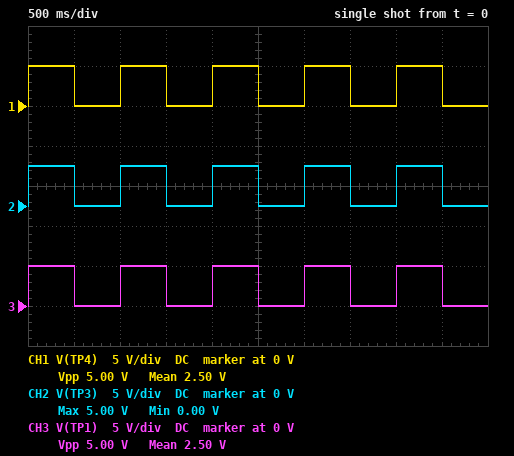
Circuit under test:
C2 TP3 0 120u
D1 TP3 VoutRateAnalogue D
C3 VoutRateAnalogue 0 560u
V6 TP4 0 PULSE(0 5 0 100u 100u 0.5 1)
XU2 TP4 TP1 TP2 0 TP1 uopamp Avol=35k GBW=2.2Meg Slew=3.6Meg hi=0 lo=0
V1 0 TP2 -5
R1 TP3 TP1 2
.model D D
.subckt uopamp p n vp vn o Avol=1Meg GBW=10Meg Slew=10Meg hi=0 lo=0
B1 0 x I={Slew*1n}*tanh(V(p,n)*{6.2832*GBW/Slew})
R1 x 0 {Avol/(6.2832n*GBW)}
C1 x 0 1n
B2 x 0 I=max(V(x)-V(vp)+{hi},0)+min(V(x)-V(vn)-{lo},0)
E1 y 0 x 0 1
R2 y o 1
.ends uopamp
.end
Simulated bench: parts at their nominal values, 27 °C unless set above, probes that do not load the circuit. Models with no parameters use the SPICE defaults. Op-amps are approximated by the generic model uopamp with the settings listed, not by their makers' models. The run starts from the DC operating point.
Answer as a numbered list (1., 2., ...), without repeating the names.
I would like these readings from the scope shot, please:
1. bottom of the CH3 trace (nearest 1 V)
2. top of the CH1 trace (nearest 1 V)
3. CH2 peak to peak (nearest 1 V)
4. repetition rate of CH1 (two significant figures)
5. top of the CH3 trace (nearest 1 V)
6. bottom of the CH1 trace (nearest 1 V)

1. 0 V
2. 5 V
3. 5 V
4. 1.0 Hz
5. 5 V
6. 0 V
